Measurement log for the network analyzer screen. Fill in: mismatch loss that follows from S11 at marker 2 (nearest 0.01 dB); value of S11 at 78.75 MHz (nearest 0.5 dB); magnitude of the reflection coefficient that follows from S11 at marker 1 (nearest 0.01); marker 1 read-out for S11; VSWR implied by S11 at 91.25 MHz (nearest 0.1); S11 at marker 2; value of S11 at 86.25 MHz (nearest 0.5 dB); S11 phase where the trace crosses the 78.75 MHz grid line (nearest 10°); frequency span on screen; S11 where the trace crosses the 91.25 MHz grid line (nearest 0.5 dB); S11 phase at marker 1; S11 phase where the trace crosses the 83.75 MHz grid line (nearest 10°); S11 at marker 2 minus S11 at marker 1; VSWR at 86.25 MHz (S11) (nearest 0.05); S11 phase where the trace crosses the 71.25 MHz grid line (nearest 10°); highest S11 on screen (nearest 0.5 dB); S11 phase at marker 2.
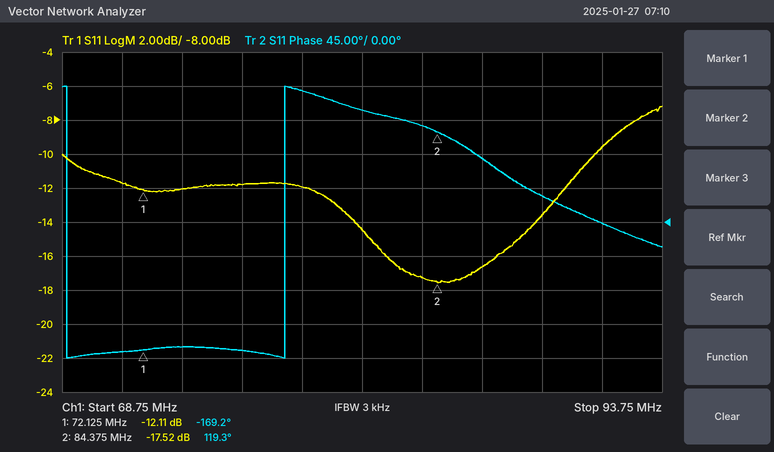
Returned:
0.08 dB
-12.0 dB
0.25
-12.11 dB
2.0
-17.52 dB
-16.5 dB
170°
25 MHz
-9.5 dB
-169.2°
130°
-5.41 dB
1.35
-170°
-7.0 dB
119.3°
